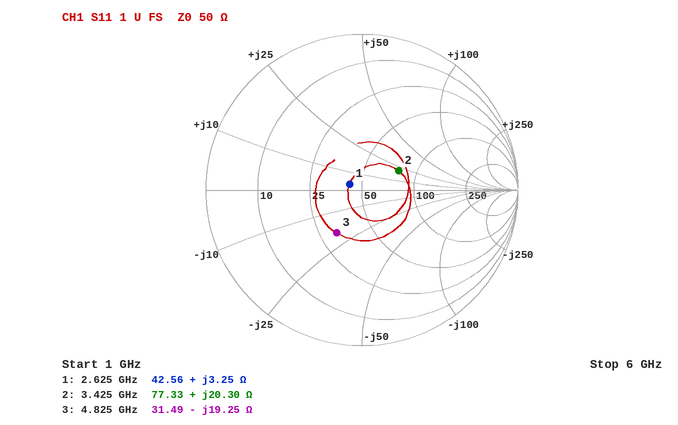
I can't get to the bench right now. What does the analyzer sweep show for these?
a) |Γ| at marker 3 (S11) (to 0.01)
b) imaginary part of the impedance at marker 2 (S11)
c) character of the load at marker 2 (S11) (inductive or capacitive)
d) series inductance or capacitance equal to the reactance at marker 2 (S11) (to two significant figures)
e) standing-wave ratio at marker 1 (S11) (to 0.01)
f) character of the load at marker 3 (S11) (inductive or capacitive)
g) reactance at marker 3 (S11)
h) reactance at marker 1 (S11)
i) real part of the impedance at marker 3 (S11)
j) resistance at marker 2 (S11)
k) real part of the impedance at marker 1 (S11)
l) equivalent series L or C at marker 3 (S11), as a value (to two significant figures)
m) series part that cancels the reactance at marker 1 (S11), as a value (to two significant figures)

0.32
+20.30 Ω
inductive
940 pH
1.19
capacitive
-19.25 Ω
+3.25 Ω
31.49 Ω
77.33 Ω
42.56 Ω
1.7 pF
19 pF
